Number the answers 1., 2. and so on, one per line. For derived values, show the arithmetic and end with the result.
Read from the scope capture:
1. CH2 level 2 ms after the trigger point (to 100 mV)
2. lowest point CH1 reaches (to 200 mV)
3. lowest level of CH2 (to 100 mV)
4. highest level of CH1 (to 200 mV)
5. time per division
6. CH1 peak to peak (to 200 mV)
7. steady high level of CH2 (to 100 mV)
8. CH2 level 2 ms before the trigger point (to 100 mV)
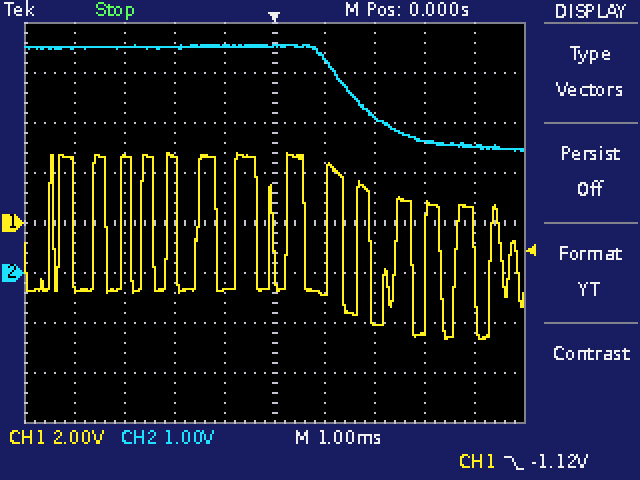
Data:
1. 3.1 V
2. -4.6 V
3. 2.4 V
4. 2.8 V
5. 1 ms
6. 2.8 V − (-4.6 V) = 7.4 V
7. 4.5 V
8. 4.5 V
